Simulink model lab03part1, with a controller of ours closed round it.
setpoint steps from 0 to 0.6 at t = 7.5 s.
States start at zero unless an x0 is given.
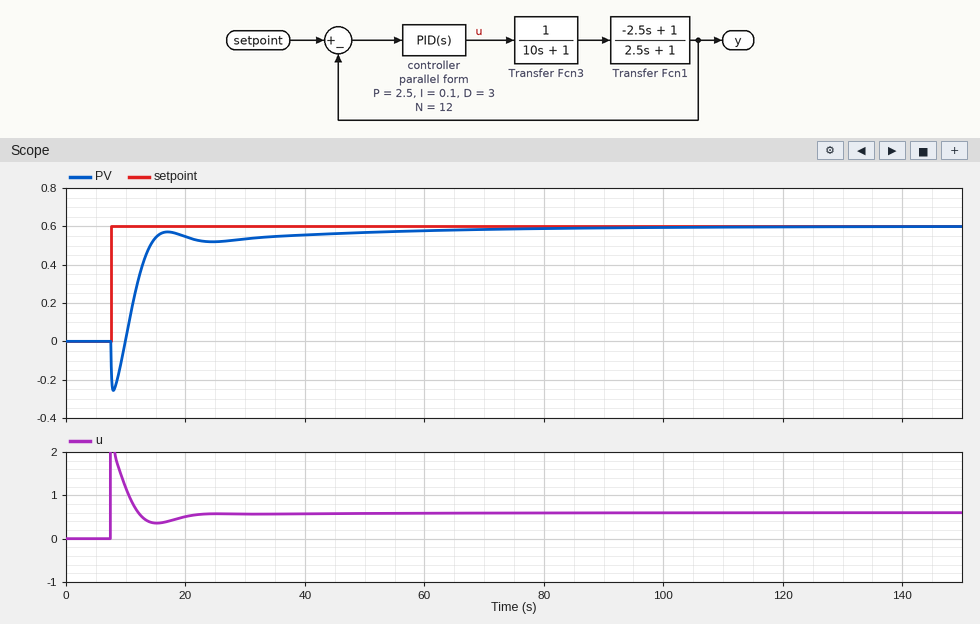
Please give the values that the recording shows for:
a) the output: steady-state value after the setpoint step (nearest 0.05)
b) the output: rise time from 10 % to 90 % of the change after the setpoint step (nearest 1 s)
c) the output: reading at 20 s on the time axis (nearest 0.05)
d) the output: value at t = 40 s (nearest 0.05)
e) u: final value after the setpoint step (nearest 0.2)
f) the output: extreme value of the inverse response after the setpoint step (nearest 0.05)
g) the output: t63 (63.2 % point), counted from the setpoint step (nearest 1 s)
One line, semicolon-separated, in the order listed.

0.60; 5 s; 0.55; 0.55; 0.6; -0.25; 5 s
